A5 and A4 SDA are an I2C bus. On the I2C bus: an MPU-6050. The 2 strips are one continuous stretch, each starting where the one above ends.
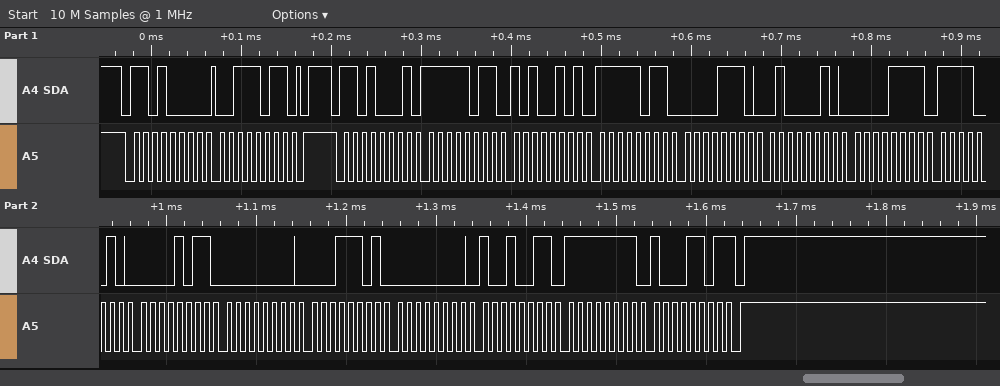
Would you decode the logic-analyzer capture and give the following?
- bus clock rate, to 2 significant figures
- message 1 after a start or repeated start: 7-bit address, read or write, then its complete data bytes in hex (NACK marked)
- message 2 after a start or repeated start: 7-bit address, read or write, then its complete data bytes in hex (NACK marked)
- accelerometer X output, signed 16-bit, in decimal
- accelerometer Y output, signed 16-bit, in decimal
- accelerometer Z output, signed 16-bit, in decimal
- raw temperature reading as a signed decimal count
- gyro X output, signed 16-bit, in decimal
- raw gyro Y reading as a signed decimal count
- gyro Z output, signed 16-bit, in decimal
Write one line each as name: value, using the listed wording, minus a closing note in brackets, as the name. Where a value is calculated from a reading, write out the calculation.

bus clock rate, to 2 significant figures: 100 kHz
message 1 after a start or repeated start: 7-bit address, read or write, then its complete data bytes in hex: 0x68 write: 3B
message 2 after a start or repeated start: 7-bit address, read or write, then its complete data bytes in hex: 0x68 read: FB A5 FB 0E 42 0F F2 0B 00 1D 00 93 FF 8D NACK
accelerometer X output, signed 16-bit, in decimal: 0xFBA5 = -1115
accelerometer Y output, signed 16-bit, in decimal: 0xFB0E = -1266
accelerometer Z output, signed 16-bit, in decimal: 0x420F = 16911
raw temperature reading as a signed decimal count: 0xF20B = -3573
gyro X output, signed 16-bit, in decimal: 0x001D = 29
raw gyro Y reading as a signed decimal count: 0x0093 = 147
gyro Z output, signed 16-bit, in decimal: 0xFF8D = -115
